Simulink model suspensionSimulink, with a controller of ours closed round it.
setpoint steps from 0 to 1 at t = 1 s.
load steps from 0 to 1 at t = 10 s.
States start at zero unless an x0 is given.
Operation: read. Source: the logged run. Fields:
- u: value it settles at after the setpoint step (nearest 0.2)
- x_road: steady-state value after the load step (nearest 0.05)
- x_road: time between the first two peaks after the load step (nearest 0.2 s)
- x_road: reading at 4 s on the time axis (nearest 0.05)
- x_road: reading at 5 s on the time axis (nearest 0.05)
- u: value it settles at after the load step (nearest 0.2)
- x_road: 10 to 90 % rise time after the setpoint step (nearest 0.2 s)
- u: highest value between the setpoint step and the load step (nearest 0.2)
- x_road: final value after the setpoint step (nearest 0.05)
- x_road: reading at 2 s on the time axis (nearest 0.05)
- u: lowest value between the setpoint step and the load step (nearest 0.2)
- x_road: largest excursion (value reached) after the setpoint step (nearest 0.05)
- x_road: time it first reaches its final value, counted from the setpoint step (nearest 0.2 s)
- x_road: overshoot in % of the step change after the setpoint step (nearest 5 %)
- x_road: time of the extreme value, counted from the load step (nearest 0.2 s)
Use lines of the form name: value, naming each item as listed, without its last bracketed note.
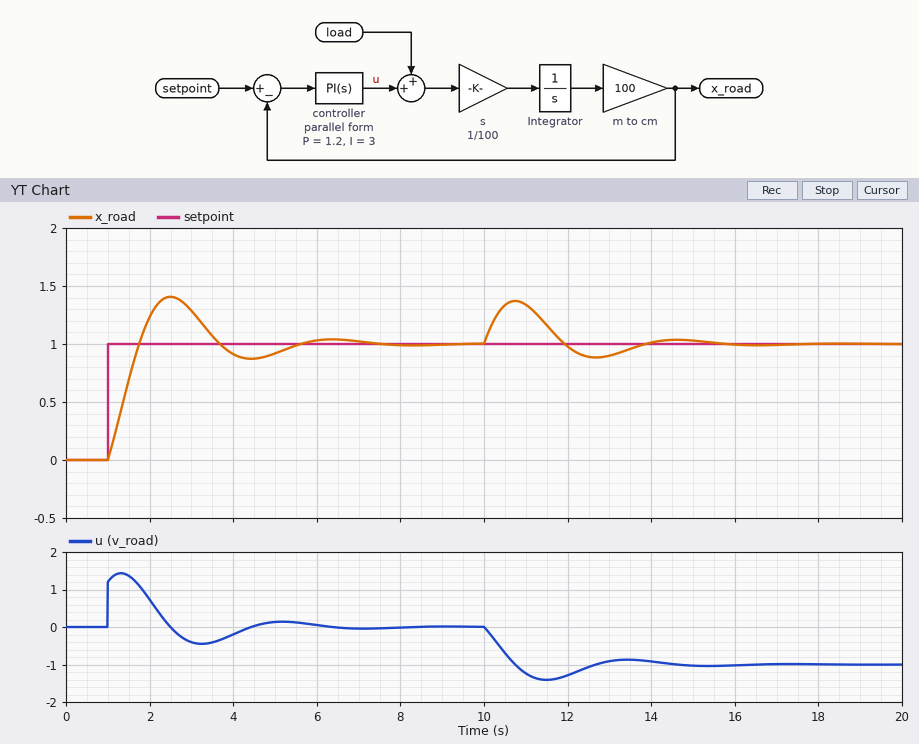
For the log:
u: value it settles at after the setpoint step: 0.0
x_road: steady-state value after the load step: 1.00
x_road: time between the first two peaks after the load step: 3.8 s
x_road: reading at 4 s on the time axis: 0.90
x_road: reading at 5 s on the time axis: 0.90
u: value it settles at after the load step: -1.0
x_road: 10 to 90 % rise time after the setpoint step: 0.6 s
u: highest value between the setpoint step and the load step: 1.4
x_road: final value after the setpoint step: 1.00
x_road: reading at 2 s on the time axis: 1.25
u: lowest value between the setpoint step and the load step: -0.4
x_road: largest excursion (value reached) after the setpoint step: 1.40
x_road: time it first reaches its final value, counted from the setpoint step: 0.8 s
x_road: overshoot in % of the step change after the setpoint step: 40 %
x_road: time of the extreme value, counted from the load step: 0.8 s
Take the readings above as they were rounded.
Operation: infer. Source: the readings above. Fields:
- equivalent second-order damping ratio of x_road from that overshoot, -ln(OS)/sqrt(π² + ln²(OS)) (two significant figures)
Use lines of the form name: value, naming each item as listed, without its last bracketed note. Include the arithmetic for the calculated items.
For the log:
equivalent second-order damping ratio of x_road from that overshoot, -ln(OS)/sqrt(π² + ln²(OS)): ln(0.4) = -0.916; 0.916 / sqrt(9.870 + 0.840) = 0.28
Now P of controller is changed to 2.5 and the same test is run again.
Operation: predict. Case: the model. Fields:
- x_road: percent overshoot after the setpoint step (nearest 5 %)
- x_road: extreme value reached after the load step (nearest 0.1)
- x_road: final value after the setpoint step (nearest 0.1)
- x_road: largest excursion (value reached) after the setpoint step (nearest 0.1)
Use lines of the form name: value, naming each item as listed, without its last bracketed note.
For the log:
x_road: percent overshoot after the setpoint step: 20 %
x_road: extreme value reached after the load step: 1.3
x_road: final value after the setpoint step: 1.0
x_road: largest excursion (value reached) after the setpoint step: 1.2
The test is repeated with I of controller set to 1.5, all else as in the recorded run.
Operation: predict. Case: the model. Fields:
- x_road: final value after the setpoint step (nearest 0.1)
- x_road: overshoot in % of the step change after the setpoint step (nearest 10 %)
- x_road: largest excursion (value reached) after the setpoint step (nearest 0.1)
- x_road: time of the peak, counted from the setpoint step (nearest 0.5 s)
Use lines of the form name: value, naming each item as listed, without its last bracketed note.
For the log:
x_road: final value after the setpoint step: 1.0
x_road: overshoot in % of the step change after the setpoint step: 30 %
x_road: largest excursion (value reached) after the setpoint step: 1.3
x_road: time of the peak, counted from the setpoint step: 2.0 s
